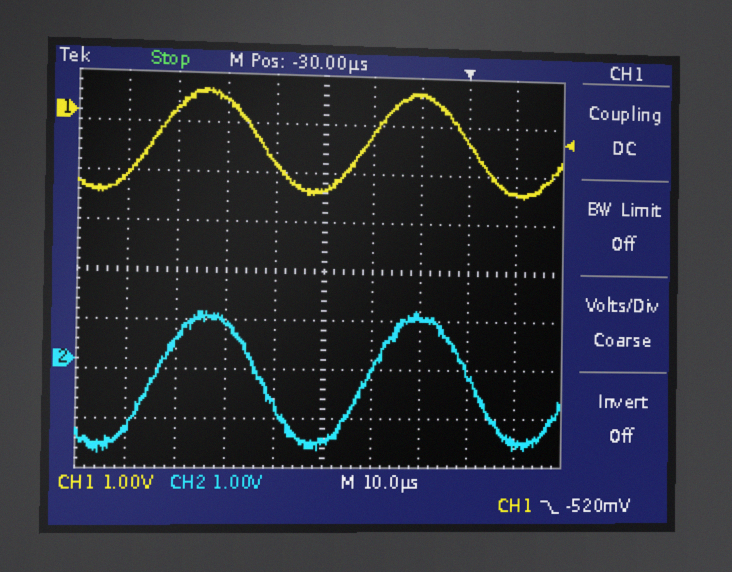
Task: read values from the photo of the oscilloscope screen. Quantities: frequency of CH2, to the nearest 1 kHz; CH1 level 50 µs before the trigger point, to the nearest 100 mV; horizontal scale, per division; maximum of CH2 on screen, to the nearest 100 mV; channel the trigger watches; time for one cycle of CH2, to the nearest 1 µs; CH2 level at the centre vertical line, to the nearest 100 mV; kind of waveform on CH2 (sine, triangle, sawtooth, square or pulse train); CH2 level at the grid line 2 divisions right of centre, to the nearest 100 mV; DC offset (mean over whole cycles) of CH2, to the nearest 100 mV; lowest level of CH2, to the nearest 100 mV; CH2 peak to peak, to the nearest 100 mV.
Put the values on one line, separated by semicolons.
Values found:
23 kHz; 300 mV; 10 µs; 1.0 V; CH1; 44 µs; -1.7 V; sine; 900 mV; -400 mV; -1.9 V; 2.9 V
